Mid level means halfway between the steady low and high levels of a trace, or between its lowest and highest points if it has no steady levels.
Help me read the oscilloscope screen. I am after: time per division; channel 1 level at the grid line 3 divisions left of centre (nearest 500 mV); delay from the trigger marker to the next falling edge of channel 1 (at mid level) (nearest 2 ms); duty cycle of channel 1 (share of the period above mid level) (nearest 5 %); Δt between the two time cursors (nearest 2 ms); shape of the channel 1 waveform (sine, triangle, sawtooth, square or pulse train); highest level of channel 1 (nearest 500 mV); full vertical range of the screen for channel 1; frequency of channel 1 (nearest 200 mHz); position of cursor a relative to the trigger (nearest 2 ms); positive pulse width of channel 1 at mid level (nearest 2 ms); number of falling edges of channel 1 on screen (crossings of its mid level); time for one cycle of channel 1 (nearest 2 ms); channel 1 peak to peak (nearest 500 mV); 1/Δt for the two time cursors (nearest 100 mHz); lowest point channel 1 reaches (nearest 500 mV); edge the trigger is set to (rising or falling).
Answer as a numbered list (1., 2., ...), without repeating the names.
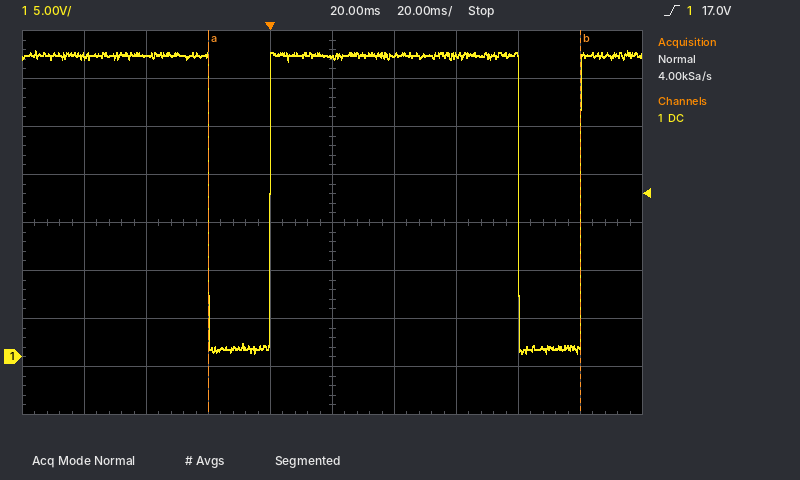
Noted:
1. 20 ms
2. 31.5 V
3. 80 ms
4. 80 %
5. 120 ms
6. pulse train
7. 32.0 V
8. 40 V
9. 10.0 Hz
10. -20 ms
11. 80 ms
12. 2
13. 100 ms
14. 31.5 V
15. 8.3 Hz
16. 500 mV
17. rising
